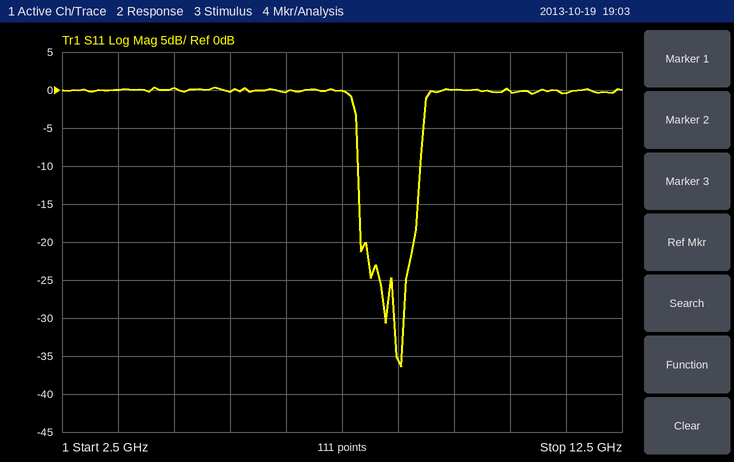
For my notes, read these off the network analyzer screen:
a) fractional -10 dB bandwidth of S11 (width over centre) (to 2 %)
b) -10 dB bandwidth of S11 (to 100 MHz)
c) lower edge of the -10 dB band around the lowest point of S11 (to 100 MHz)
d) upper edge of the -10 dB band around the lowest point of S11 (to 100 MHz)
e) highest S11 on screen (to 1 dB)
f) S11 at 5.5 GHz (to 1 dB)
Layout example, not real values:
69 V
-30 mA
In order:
14 %
1.1 GHz
7.8 GHz
8.9 GHz
0 dB
0 dB
